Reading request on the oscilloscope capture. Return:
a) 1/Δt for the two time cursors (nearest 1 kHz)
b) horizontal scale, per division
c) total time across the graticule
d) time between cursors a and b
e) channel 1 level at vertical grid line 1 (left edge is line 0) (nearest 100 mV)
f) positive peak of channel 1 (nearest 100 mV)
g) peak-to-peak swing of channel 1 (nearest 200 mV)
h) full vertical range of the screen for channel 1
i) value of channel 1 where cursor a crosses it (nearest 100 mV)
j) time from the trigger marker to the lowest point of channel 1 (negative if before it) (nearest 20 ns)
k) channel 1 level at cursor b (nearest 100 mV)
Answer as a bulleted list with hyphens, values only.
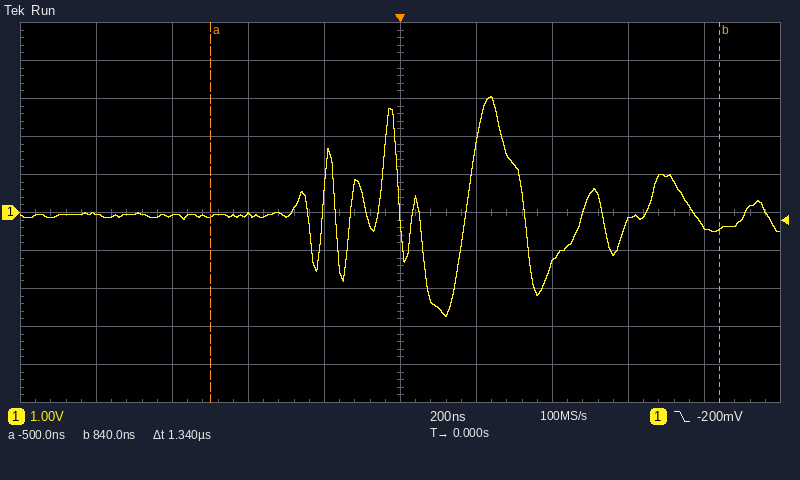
- 746 kHz
- 200 ns
- 2 µs
- 1.34 µs
- 0.0 V
- 3.1 V
- 5.8 V
- 10 V
- -100 mV
- +120 ns
- -400 mV
